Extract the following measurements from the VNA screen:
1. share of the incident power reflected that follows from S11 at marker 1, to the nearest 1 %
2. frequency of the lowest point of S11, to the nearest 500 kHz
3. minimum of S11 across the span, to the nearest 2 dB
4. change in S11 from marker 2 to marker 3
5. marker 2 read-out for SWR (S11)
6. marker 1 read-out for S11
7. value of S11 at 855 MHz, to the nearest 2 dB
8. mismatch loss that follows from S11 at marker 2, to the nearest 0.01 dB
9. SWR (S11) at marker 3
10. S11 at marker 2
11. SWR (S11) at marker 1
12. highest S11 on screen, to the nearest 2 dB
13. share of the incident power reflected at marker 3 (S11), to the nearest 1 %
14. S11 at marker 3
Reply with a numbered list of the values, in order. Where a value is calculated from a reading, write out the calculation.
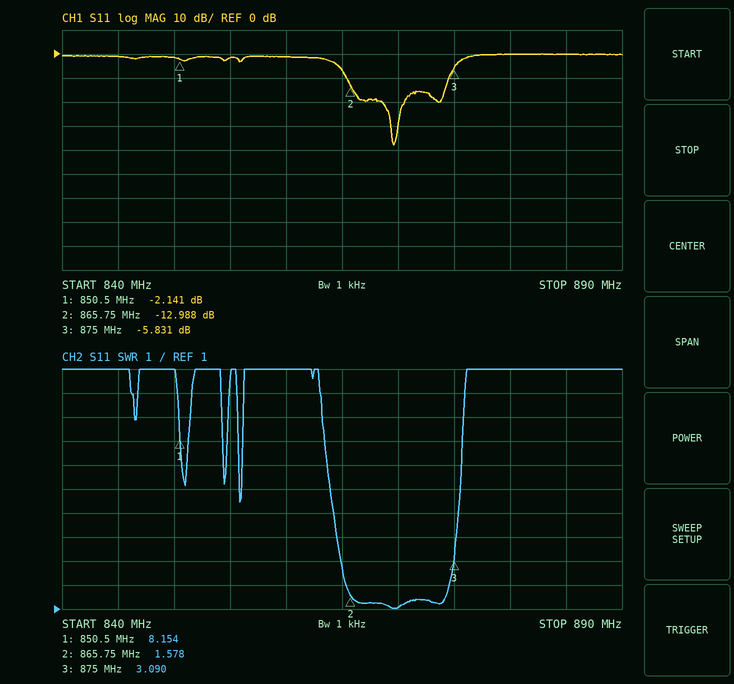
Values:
1. 10^(-2.141/10) ≈ 61 %
2. 869.5 MHz
3. -38 dB
4. -5.831 − (-12.988) = 7.157 dB
5. 1.578
6. -2.141 dB
7. -2 dB
8. −10 log10(1 − 10^(-12.988/10)) ≈ 0.22 dB
9. 3.090
10. -12.988 dB
11. 8.154
12. 0 dB
13. 10^(-5.831/10) ≈ 26 %
14. -5.831 dB
